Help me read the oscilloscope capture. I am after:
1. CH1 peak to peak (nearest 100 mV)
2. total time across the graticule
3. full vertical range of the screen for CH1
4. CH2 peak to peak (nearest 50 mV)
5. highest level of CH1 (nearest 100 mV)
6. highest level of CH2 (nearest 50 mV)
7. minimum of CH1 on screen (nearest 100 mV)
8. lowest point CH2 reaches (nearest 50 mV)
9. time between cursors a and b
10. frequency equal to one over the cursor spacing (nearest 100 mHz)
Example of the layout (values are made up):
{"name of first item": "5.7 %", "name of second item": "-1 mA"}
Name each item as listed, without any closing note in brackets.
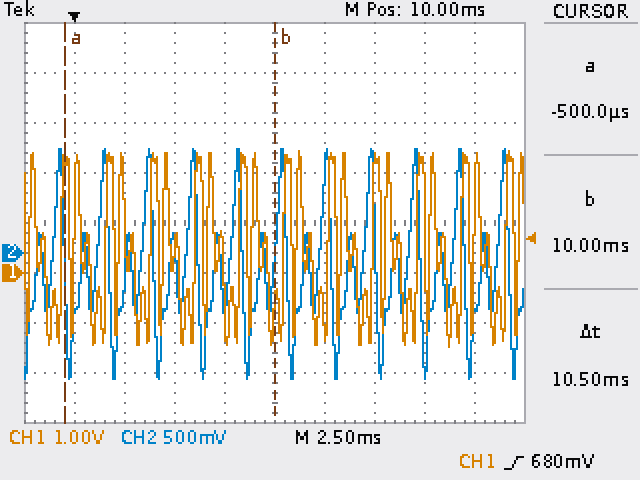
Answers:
{"CH1 peak to peak": "3.9 V", "total time across the graticule": "25 ms", "full vertical range of the screen for CH1": "8 V", "CH2 peak to peak": "2.30 V", "highest level of CH1": "2.4 V", "highest level of CH2": "1.05 V", "minimum of CH1 on screen": "-1.5 V", "lowest point CH2 reaches": "-1.25 V", "time between cursors a and b": "10.5 ms", "frequency equal to one over the cursor spacing": "95.2 Hz"}
